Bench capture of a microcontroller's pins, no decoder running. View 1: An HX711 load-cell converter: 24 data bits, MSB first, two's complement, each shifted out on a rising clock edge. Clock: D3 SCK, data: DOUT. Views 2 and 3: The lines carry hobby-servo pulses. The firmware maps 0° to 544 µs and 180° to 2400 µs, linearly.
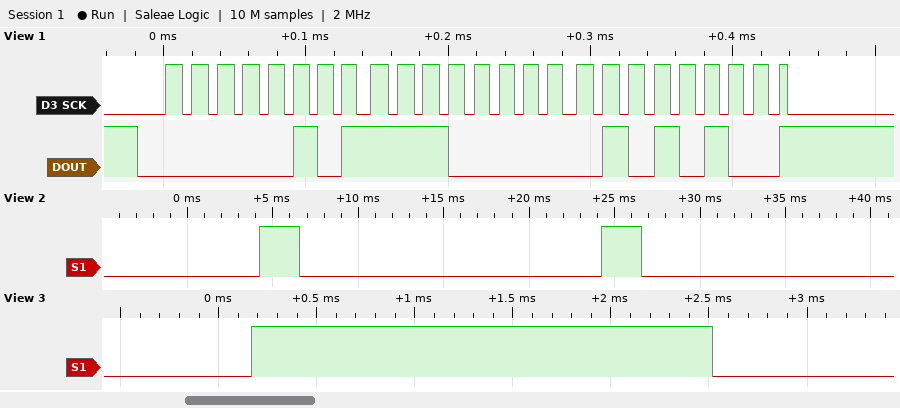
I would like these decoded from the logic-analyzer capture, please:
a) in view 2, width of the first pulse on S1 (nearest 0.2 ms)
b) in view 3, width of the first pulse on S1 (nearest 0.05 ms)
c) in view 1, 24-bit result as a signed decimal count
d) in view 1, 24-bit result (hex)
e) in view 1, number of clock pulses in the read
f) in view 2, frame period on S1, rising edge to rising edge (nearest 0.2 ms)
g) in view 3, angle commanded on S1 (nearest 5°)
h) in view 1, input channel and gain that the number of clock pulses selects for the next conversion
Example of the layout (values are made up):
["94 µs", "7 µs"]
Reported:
["2.4 ms", "2.35 ms", "385108", "0x05E054", "25", "20.0 ms", "175°", "channel A, gain 128"]
